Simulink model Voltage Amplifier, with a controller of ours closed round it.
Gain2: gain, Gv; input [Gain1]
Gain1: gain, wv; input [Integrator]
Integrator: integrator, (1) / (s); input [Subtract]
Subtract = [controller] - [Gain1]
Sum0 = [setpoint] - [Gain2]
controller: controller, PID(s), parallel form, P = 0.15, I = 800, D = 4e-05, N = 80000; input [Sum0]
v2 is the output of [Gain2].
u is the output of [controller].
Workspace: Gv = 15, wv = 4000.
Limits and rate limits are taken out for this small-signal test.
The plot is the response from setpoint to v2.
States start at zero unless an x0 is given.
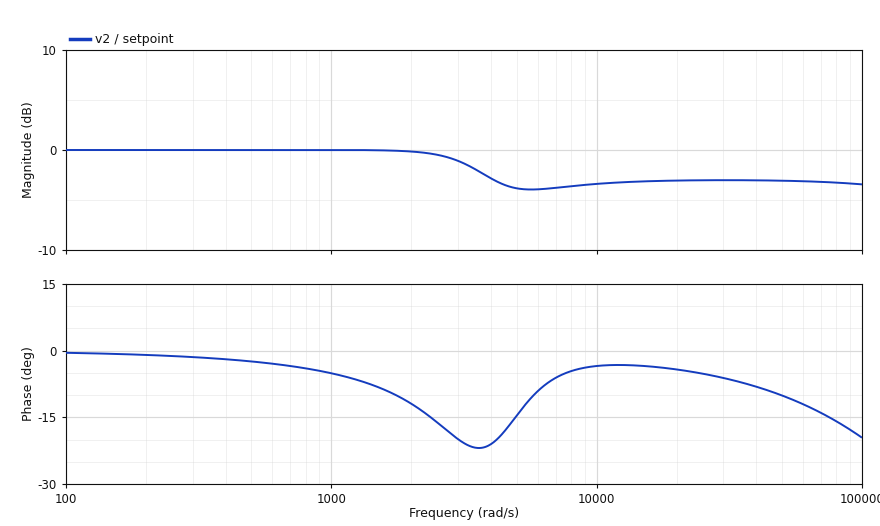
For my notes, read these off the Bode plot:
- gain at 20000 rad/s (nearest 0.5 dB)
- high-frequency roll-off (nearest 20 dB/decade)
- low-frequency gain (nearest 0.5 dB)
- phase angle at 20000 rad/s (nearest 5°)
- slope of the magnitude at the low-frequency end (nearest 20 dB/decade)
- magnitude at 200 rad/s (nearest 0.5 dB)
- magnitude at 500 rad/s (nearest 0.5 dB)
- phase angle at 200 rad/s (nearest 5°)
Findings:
-3.0 dB
0 dB/decade
0.0 dB
-5°
0 dB/decade
0.0 dB
0.0 dB
0°
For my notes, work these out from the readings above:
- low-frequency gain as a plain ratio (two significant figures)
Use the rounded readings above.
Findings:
1.0
